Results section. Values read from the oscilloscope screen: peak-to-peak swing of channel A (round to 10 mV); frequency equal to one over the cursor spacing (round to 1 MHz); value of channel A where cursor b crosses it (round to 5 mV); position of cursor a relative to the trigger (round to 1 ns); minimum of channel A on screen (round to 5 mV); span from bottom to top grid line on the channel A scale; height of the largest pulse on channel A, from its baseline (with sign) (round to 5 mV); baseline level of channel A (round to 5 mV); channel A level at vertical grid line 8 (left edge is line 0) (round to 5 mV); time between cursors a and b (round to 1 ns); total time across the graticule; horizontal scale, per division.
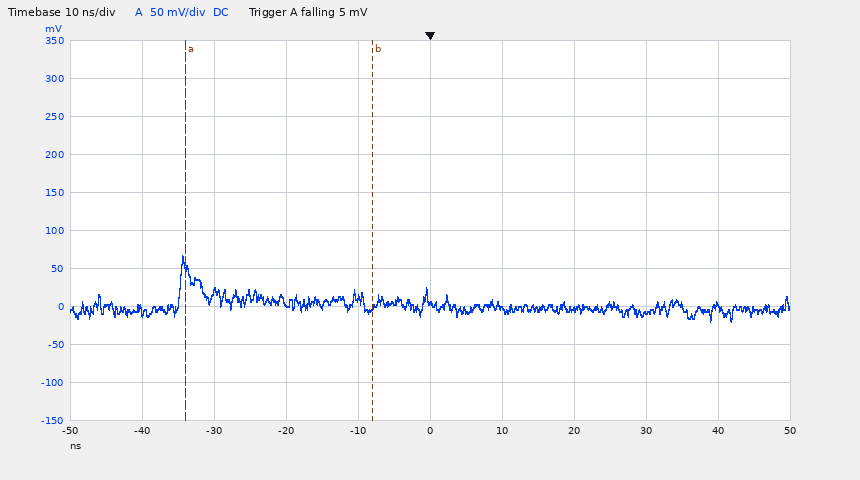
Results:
90 mV
38 MHz
0 mV
-34 ns
-20 mV
500 mV
+70 mV
0 mV
-10 mV
26 ns
100 ns
10 ns
